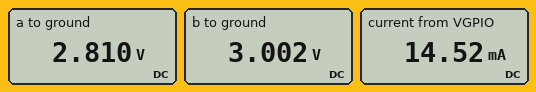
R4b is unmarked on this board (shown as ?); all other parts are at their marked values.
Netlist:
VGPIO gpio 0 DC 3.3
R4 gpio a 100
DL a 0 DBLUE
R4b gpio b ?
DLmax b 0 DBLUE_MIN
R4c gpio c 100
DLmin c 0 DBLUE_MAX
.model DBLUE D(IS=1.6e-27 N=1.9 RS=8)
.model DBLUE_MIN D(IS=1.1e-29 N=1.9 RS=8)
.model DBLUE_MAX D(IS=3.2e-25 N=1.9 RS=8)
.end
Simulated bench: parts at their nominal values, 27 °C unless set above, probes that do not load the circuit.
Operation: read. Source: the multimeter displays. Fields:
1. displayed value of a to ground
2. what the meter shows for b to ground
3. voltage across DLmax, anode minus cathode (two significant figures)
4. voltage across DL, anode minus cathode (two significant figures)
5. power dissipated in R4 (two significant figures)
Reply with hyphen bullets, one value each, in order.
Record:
- 2.810 V
- 3.002 V
- 3.0 V
- 2.8 V
- 2.4 mW
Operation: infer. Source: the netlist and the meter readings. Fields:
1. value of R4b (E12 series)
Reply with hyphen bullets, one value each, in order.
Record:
- 120 Ω
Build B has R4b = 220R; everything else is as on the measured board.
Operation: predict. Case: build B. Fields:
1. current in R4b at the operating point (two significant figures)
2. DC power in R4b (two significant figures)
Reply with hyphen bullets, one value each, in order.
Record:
- 1.5 mA
- 500 µW
